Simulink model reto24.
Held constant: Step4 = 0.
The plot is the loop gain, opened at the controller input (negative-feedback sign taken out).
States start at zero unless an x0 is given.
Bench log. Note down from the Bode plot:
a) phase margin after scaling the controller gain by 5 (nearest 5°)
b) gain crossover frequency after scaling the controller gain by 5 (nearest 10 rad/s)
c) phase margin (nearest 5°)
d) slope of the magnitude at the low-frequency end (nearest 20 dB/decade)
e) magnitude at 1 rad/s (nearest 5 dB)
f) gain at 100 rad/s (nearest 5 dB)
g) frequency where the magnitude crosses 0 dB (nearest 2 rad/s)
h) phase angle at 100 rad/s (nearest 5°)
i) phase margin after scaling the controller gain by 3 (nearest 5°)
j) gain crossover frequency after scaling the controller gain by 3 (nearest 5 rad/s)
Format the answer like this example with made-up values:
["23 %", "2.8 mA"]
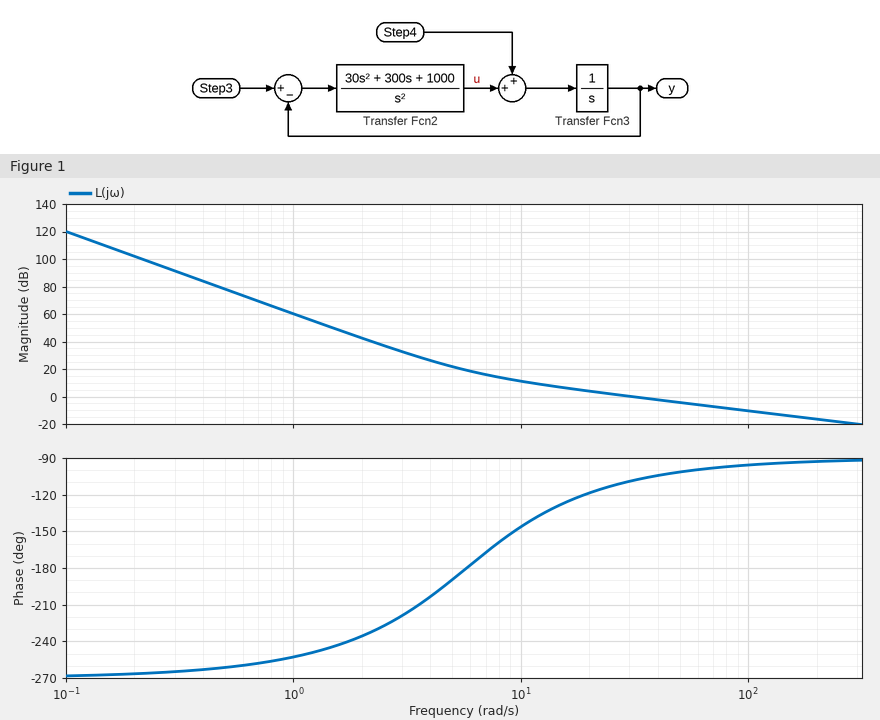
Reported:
["85°", "150 rad/s", "70°", "-60 dB/decade", "60 dB", "-10 dB", "30 rad/s", "-95°", "85°", "90 rad/s"]
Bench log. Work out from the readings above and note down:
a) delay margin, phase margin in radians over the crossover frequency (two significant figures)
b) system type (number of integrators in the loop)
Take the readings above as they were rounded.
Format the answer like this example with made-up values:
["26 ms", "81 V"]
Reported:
["0.041 s", "3"]
